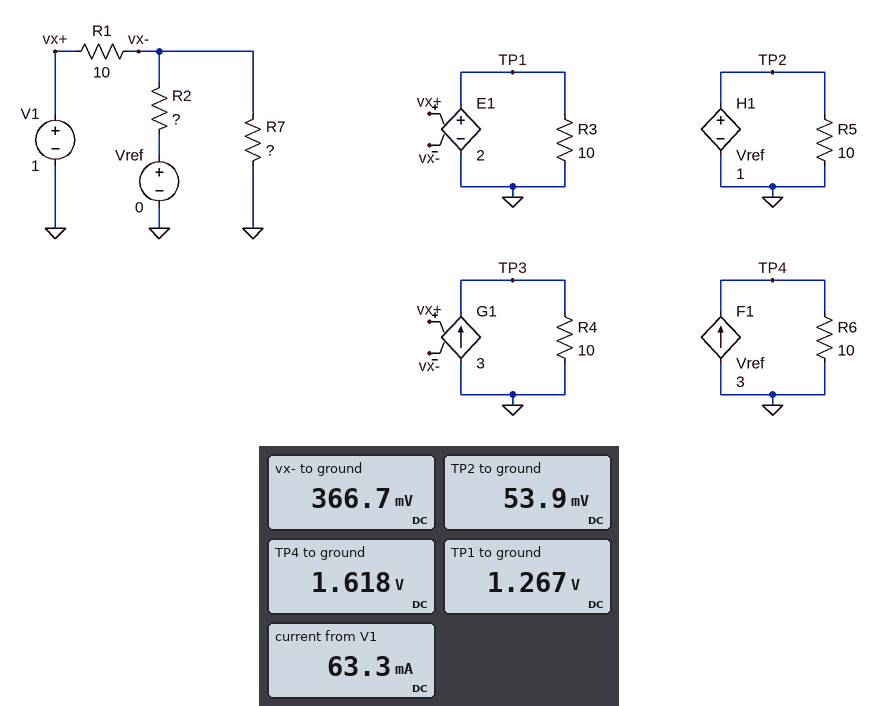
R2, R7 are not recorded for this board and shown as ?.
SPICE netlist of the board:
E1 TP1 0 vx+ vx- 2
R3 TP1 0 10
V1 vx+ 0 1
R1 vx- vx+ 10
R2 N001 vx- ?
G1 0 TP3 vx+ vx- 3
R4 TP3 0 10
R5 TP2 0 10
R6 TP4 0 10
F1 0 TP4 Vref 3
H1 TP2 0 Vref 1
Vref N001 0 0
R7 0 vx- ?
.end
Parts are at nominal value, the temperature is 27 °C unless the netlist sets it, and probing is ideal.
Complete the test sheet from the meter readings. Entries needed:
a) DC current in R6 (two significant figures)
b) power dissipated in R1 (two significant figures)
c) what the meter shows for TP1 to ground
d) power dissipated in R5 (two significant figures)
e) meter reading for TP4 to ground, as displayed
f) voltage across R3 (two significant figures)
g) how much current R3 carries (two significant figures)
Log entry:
160 mA
40 mW
1.267 V
290 µW
1.618 V
1.3 V
130 mA
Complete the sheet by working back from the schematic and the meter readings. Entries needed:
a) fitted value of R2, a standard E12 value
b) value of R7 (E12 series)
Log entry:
6.8 Ω
39 Ω
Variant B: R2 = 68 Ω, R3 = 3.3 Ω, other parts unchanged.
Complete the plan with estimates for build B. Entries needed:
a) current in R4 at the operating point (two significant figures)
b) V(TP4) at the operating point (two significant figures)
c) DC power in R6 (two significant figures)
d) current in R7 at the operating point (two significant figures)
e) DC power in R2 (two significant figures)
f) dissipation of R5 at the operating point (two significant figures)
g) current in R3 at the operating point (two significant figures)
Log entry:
860 mA
310 mV
9.9 mW
18 mA
7.5 mW
11 µW
170 mA
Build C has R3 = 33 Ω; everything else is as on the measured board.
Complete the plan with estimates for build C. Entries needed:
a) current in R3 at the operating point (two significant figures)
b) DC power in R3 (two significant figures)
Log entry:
38 mA
49 mW
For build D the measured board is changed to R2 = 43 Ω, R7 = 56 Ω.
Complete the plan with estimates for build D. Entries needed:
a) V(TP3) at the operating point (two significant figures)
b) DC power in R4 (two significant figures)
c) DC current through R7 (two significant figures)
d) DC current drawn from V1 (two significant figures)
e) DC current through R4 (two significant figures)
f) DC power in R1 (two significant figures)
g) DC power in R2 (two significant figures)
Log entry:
8.7 V
7.6 W
13 mA
29 mA
870 mA
8.5 mW
12 mW
